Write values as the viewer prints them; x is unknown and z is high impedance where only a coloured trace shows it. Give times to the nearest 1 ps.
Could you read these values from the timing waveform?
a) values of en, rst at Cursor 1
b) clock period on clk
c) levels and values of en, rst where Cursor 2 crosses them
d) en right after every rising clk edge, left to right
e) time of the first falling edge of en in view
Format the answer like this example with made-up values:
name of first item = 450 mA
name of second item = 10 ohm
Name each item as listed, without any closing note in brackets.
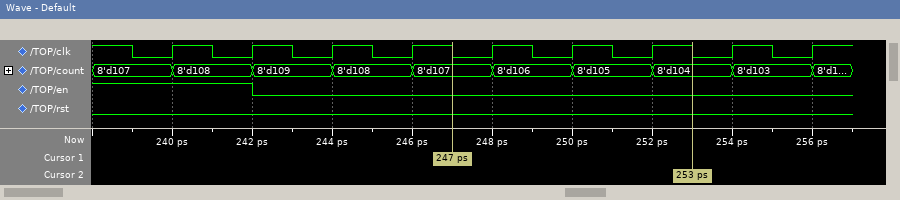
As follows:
values of en, rst at Cursor 1 = en=0, rst=0
clock period on clk = 2 ps
levels and values of en, rst where Cursor 2 crosses them = en=0, rst=0
en right after every rising clk edge, left to right = 1 0 0 0 0 0 0 0 0
time of the first falling edge of en in view = 242 ps
